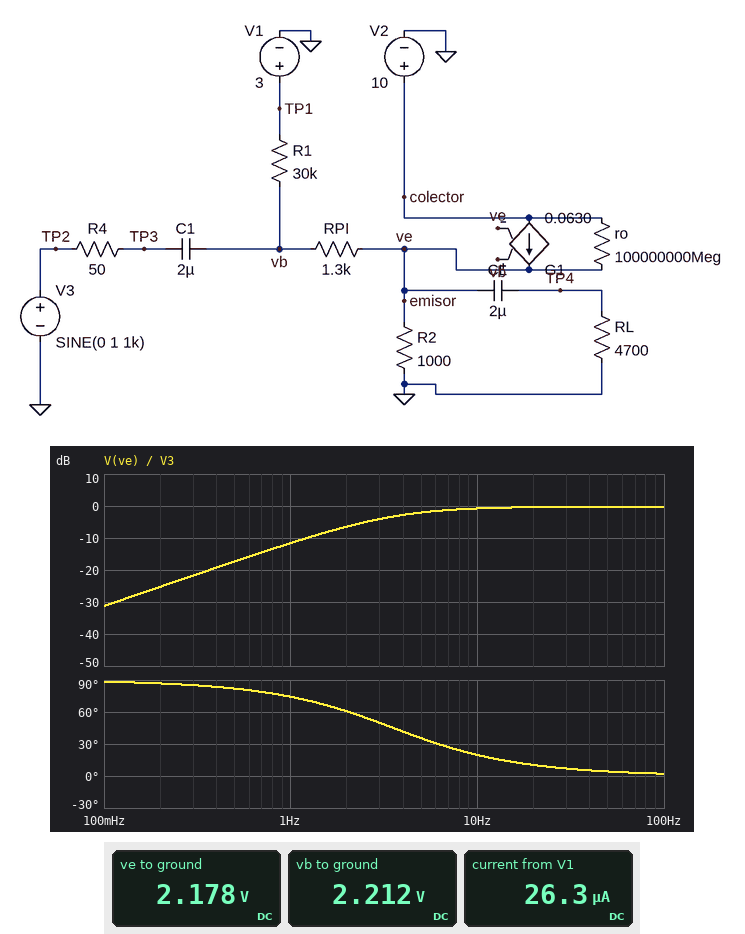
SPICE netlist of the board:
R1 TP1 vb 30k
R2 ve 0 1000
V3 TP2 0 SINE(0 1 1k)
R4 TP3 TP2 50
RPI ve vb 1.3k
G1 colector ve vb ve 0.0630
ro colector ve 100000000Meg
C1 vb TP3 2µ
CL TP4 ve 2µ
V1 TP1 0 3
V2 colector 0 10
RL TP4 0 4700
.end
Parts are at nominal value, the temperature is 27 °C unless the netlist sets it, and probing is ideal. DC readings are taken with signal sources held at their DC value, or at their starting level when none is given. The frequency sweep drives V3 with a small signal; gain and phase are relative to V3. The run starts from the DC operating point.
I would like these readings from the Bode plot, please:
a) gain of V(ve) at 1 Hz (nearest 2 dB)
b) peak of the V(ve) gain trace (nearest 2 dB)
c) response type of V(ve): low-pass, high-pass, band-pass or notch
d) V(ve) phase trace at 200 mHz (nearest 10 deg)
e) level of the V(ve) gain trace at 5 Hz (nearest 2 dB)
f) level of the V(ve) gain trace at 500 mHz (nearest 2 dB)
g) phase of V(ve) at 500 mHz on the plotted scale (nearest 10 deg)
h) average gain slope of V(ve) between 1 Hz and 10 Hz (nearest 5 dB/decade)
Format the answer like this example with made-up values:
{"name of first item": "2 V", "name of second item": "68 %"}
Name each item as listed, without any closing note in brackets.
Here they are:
{"gain of V(ve) at 1 Hz": "-12 dB", "peak of the V(ve) gain trace": "0 dB", "response type of V(ve): low-pass, high-pass, band-pass or notch": "high-pass", "V(ve) phase trace at 200 mHz": "90 deg", "level of the V(ve) gain trace at 5 Hz": "-2 dB", "level of the V(ve) gain trace at 500 mHz": "-18 dB", "phase of V(ve) at 500 mHz on the plotted scale": "80 deg", "average gain slope of V(ve) between 1 Hz and 10 Hz": "10 dB/decade"}
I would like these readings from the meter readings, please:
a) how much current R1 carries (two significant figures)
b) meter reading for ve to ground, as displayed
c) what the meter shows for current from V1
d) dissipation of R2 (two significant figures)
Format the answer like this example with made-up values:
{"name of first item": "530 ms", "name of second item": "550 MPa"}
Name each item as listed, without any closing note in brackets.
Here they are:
{"how much current R1 carries": "26 µA", "meter reading for ve to ground, as displayed": "2.178 V", "what the meter shows for current from V1": "26.3 µA", "dissipation of R2": "4.7 mW"}
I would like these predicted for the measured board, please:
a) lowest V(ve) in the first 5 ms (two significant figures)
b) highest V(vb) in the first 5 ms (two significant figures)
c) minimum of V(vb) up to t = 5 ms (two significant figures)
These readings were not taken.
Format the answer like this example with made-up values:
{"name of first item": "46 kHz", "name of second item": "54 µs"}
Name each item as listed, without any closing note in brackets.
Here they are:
{"lowest V(ve) in the first 5 ms": "1.2 V", "highest V(vb) in the first 5 ms": "3.2 V", "minimum of V(vb) up to t = 5 ms": "1.2 V"}
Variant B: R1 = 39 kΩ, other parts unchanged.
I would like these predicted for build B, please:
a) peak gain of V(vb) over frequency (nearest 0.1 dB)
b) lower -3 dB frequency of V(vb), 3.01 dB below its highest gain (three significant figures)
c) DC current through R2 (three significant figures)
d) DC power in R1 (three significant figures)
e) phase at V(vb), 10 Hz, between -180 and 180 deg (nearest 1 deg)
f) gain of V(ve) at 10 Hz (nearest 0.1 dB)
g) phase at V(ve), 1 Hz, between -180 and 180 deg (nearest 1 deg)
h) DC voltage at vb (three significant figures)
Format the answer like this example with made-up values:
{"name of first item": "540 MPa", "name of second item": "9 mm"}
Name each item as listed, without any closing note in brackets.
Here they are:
{"peak gain of V(vb) over frequency": "0 dB", "lower -3 dB frequency of V(vb), 3.01 dB below its highest gain": "3.02 Hz", "DC current through R2": "2.02 mA", "DC power in R1": "23.1 µW", "phase at V(vb), 10 Hz, between -180 and 180 deg": "17 deg", "gain of V(ve) at 10 Hz": "-0.6 dB", "phase at V(ve), 1 Hz, between -180 and 180 deg": "71 deg", "DC voltage at vb": "2.05 V"}
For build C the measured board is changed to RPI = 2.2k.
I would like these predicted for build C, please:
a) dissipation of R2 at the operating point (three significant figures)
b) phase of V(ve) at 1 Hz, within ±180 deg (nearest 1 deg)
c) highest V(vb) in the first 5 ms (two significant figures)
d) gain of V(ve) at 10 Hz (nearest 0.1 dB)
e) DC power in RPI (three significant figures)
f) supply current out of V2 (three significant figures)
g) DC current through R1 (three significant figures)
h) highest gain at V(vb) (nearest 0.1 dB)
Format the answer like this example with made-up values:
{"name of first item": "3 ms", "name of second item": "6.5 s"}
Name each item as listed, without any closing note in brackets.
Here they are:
{"dissipation of R2 at the operating point": "5.94 mW", "phase of V(ve) at 1 Hz, within ±180 deg": "73 deg", "highest V(vb) in the first 5 ms": "3.5 V", "gain of V(ve) at 10 Hz": "-0.6 dB", "DC power in RPI": "671 nW", "supply current out of V2": "2.42 mA", "DC current through R1": "17.5 µA", "highest gain at V(vb)": "0 dB"}
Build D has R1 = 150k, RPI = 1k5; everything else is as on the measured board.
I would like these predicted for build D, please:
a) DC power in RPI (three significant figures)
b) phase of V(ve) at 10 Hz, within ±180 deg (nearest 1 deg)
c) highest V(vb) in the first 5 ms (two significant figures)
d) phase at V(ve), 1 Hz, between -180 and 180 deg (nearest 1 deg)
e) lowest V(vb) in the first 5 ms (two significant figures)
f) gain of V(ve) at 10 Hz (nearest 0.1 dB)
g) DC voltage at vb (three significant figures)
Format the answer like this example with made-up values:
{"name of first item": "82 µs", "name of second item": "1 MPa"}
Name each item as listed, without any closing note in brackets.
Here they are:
{"DC power in RPI": "221 nW", "phase of V(ve) at 10 Hz, within ±180 deg": "8 deg", "highest V(vb) in the first 5 ms": "2.2 V", "phase at V(ve), 1 Hz, between -180 and 180 deg": "53 deg", "lowest V(vb) in the first 5 ms": "180 mV", "gain of V(ve) at 10 Hz": "-0.3 dB", "DC voltage at vb": "1.18 V"}
